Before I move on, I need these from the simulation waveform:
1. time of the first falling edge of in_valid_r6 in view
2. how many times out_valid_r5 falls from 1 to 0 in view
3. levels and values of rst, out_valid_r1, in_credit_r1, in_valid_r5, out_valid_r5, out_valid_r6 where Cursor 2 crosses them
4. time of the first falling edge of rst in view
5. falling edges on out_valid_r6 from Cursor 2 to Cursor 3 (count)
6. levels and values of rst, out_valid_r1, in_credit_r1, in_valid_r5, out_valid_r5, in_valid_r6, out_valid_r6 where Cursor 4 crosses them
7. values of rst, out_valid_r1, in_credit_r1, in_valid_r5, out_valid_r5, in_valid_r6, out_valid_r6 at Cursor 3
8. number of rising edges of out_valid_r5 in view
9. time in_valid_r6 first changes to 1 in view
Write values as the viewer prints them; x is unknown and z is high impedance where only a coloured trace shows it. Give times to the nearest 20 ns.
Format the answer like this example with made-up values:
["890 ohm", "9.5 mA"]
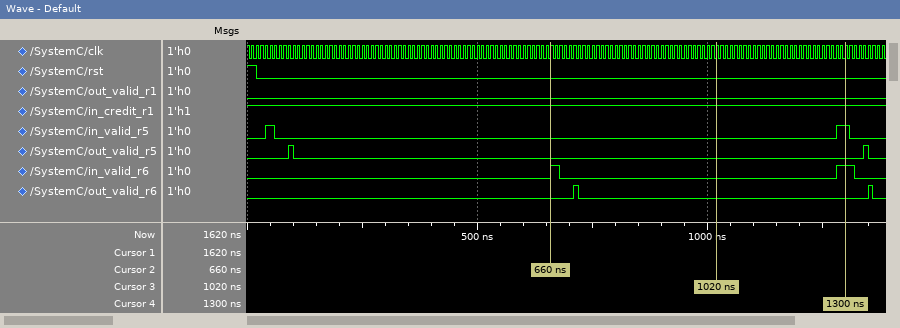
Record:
["680 ns", "2", "rst=0, out_valid_r1=0, in_credit_r1=1, in_valid_r5=0, out_valid_r5=0, out_valid_r6=0", "20 ns", "1", "rst=0, out_valid_r1=0, in_credit_r1=1, in_valid_r5=1, out_valid_r5=0, in_valid_r6=1, out_valid_r6=0", "rst=0, out_valid_r1=0, in_credit_r1=1, in_valid_r5=0, out_valid_r5=0, in_valid_r6=0, out_valid_r6=0", "2", "660 ns"]
